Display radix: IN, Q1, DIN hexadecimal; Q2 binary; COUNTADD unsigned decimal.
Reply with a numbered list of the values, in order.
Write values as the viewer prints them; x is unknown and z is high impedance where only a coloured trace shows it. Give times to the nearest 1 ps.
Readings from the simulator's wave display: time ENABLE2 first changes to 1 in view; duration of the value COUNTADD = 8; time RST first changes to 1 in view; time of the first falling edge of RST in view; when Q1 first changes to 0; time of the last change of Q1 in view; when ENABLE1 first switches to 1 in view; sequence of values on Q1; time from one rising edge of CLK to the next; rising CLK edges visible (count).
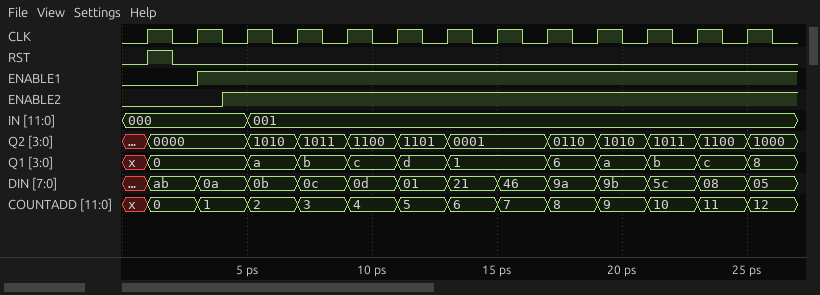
1. 4 ps
2. 2 ps
3. 1 ps
4. 2 ps
5. 1 ps
6. 25 ps
7. 3 ps
8. x, 0, a, b, c, d, 1, 6, a, b, c, 8
9. 2 ps
10. 13
